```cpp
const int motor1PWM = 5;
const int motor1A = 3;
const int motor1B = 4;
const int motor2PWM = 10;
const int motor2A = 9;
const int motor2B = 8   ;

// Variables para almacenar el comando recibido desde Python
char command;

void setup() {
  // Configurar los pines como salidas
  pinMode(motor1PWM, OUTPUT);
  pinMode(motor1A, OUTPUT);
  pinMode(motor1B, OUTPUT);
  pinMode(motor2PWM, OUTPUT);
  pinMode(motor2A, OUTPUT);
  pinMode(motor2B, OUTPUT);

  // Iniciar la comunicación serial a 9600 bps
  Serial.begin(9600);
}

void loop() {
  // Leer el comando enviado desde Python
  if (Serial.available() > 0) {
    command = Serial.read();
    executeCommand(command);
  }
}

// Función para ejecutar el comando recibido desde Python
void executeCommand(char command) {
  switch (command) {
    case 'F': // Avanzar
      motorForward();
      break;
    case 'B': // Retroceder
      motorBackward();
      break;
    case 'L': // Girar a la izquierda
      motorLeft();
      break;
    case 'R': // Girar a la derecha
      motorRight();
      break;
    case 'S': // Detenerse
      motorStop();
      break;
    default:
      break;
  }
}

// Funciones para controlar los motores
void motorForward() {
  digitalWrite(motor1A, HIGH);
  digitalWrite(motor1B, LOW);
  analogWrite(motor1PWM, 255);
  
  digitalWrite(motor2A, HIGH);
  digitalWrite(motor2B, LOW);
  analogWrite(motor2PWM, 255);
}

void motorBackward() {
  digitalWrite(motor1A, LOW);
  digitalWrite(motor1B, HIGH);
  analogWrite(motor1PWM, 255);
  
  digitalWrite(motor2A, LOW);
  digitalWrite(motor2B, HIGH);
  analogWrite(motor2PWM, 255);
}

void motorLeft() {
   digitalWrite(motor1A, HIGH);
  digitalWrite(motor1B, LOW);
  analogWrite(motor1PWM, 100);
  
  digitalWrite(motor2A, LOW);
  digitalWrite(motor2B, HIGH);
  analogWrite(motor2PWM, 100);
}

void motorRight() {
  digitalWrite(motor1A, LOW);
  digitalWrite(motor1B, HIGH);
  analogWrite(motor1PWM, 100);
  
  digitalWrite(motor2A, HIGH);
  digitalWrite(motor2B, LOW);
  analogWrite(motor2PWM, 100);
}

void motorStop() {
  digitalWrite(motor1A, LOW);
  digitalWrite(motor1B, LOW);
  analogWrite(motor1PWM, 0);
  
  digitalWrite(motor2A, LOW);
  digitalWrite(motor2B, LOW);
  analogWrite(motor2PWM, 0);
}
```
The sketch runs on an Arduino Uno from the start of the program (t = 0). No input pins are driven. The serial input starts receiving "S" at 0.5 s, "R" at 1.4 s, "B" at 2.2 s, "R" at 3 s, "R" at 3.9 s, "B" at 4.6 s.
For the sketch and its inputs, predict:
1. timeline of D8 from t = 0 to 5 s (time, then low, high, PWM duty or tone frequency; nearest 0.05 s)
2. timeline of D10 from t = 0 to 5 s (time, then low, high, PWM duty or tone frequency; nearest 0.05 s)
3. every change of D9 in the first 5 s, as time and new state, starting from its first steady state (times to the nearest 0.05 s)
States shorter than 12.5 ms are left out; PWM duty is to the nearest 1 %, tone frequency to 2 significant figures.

0 s low; 2.2 s high; 3 s low; 4.6 s high
0 s low; 1.4 s PWM 39 %; 2.2 s high; 3 s PWM 39 %; 4.6 s high
0 s low; 1.4 s high; 2.2 s low; 3 s high; 4.6 s low
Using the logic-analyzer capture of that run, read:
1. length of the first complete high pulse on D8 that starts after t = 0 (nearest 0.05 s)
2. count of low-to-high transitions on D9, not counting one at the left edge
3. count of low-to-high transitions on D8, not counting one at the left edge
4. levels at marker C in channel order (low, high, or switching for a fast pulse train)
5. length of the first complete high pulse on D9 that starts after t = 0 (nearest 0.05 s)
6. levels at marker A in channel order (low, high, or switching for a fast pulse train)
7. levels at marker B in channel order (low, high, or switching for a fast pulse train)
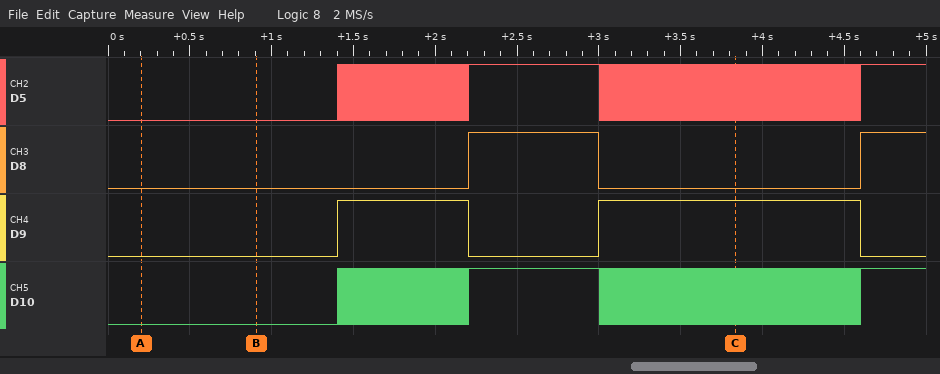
0.80 s
2
2
D5 switching, D8 low, D9 high, D10 switching
0.80 s
D5 low, D8 low, D9 low, D10 low
D5 low, D8 low, D9 low, D10 low
